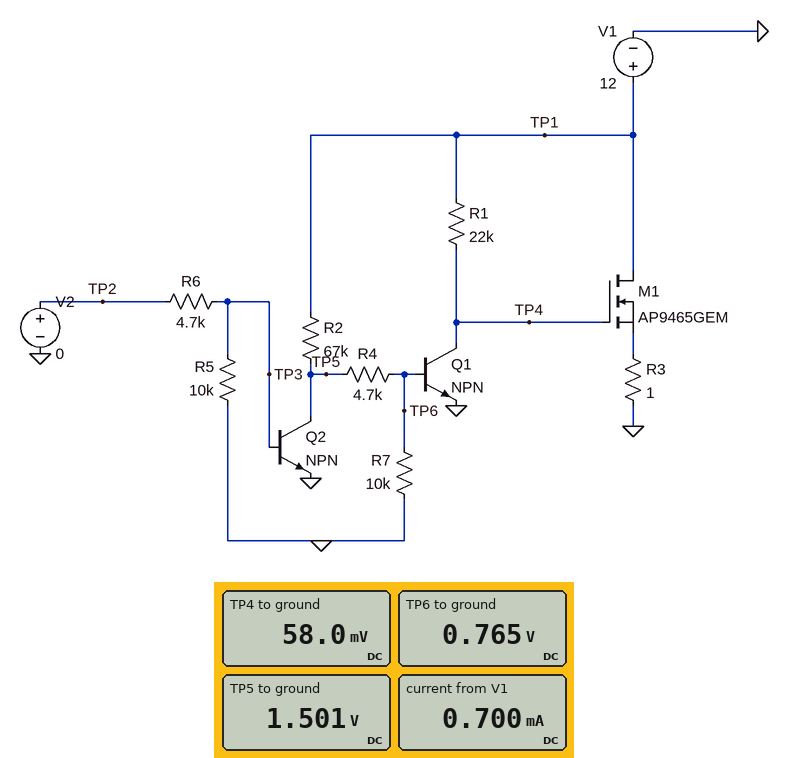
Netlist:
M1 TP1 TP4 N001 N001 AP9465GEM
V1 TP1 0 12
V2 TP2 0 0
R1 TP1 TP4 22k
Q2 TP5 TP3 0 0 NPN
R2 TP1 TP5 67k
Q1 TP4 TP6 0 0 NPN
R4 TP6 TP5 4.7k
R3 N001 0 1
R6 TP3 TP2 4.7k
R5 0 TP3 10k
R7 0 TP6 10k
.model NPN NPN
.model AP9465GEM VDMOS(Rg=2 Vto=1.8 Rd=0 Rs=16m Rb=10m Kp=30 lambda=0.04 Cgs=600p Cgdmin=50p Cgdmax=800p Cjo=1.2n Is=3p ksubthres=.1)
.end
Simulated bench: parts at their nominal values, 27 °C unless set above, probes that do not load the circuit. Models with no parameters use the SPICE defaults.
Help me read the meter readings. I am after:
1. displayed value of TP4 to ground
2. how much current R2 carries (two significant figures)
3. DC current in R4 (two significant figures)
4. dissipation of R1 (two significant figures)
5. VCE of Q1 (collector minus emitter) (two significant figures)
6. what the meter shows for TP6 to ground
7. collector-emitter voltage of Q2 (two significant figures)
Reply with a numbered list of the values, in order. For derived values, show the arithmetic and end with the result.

1. 58.0 mV
2. (12 V - 1.501 V) / 67 kΩ = 160 µA
3. (1.501 V - 765 mV) / 4.7 kΩ = 160 µA
4. (12 V - 58 mV)^2 / 22 kΩ = 6.5 mW
5. 58 mV = 58 mV
6. 0.765 V
7. 1.501 V = 1.5 V
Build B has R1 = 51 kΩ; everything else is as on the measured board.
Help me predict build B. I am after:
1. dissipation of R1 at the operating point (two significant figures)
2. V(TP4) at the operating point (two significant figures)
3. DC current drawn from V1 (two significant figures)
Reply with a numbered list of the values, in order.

1. 2.8 mW
2. 42 mV
3. 390 µA
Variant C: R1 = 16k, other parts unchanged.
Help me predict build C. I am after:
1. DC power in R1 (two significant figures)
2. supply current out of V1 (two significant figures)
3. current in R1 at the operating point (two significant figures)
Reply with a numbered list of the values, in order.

1. 8.9 mW
2. 900 µA
3. 750 µA
